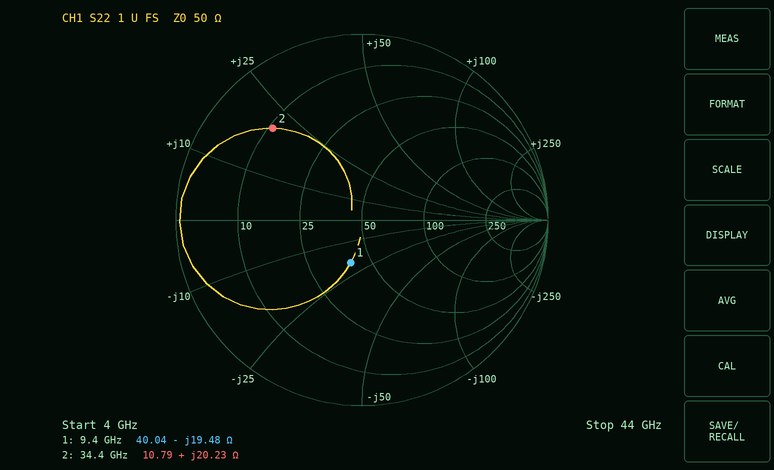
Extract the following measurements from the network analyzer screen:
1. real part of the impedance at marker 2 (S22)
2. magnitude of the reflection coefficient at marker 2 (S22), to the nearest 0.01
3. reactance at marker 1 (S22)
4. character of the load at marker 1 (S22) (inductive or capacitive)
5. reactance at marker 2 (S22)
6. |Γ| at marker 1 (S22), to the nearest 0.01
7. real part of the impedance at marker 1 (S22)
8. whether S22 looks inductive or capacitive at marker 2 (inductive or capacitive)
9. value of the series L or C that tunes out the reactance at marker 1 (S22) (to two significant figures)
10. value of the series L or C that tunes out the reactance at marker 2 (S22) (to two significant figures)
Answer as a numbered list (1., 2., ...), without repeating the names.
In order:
1. 10.79 Ω
2. 0.69
3. -19.48 Ω
4. capacitive
5. +20.23 Ω
6. 0.24
7. 40.04 Ω
8. inductive
9. 330 pH
10. 230 fF
